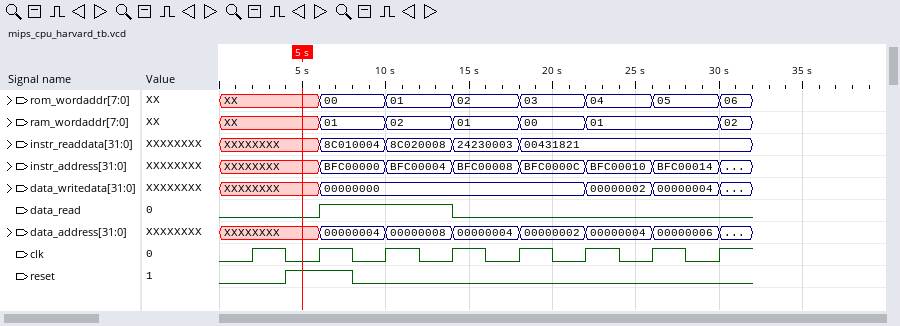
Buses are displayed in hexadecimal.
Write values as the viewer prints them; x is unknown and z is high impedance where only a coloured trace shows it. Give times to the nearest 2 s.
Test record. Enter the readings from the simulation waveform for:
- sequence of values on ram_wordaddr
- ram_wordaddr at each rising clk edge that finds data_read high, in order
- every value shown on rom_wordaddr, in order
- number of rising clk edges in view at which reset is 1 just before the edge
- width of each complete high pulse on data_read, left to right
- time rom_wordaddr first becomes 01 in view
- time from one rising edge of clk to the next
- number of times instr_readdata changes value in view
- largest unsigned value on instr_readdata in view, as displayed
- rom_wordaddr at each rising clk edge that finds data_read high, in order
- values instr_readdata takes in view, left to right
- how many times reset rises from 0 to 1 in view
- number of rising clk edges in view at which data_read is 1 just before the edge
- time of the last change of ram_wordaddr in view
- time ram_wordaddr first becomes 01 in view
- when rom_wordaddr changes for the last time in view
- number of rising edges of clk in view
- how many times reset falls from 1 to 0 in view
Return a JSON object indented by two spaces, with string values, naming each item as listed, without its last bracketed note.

{
  "sequence of values on ram_wordaddr": "XX, 01, 02, 01, 00, 01, 02",
  "ram_wordaddr at each rising clk edge that finds data_read high, in order": "01, 02",
  "every value shown on rom_wordaddr, in order": "XX, 00, 01, 02, 03, 04, 05, 06",
  "number of rising clk edges in view at which reset is 1 just before the edge": "1",
  "width of each complete high pulse on data_read, left to right": "8 s",
  "time rom_wordaddr first becomes 01 in view": "10 s",
  "time from one rising edge of clk to the next": "4 s",
  "number of times instr_readdata changes value in view": "4",
  "largest unsigned value on instr_readdata in view, as displayed": "8C020008",
  "rom_wordaddr at each rising clk edge that finds data_read high, in order": "00, 01",
  "values instr_readdata takes in view, left to right": "XXXXXXXX, 8C010004, 8C020008, 24230003, 00431821",
  "how many times reset rises from 0 to 1 in view": "1",
  "number of rising clk edges in view at which data_read is 1 just before the edge": "2",
  "time of the last change of ram_wordaddr in view": "30 s",
  "time ram_wordaddr first becomes 01 in view": "6 s",
  "when rom_wordaddr changes for the last time in view": "30 s",
  "number of rising edges of clk in view": "8",
  "how many times reset falls from 1 to 0 in view": "1"
}
